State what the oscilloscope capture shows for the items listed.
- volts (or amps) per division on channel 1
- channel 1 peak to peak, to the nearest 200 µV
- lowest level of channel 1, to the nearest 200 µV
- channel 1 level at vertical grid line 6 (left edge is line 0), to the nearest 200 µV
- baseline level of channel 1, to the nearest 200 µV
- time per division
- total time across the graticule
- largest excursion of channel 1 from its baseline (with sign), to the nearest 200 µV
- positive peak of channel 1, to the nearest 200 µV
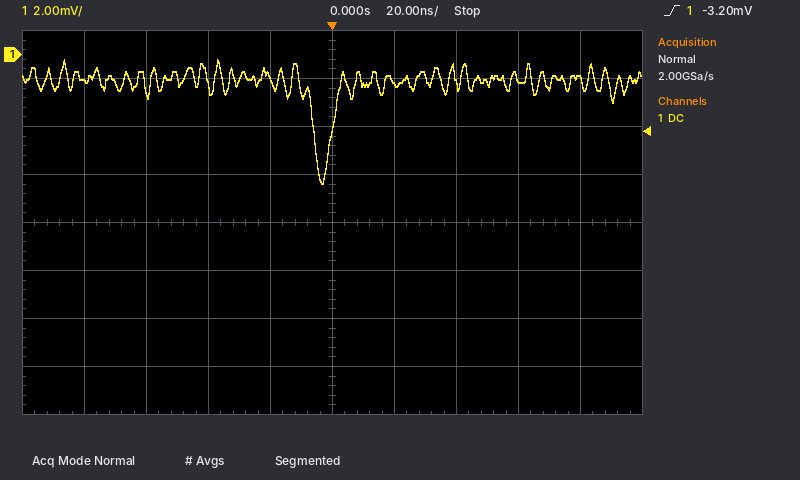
2 mV
5.2 mV
-5.4 mV
-1.2 mV
-1.0 mV
20 ns
200 ns
-4.4 mV
-200 µV
